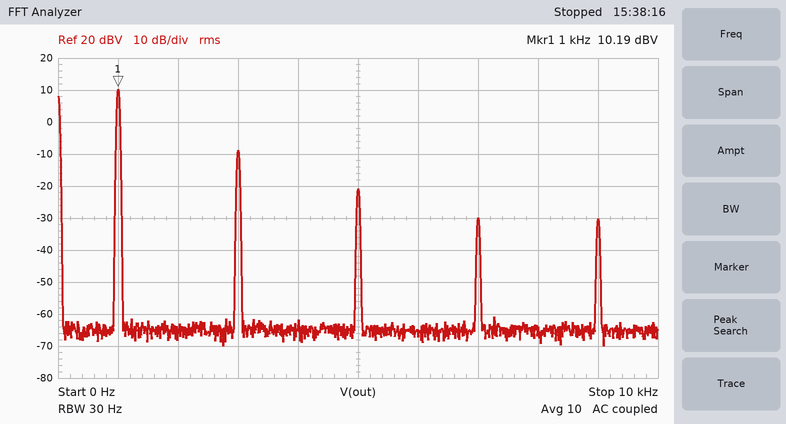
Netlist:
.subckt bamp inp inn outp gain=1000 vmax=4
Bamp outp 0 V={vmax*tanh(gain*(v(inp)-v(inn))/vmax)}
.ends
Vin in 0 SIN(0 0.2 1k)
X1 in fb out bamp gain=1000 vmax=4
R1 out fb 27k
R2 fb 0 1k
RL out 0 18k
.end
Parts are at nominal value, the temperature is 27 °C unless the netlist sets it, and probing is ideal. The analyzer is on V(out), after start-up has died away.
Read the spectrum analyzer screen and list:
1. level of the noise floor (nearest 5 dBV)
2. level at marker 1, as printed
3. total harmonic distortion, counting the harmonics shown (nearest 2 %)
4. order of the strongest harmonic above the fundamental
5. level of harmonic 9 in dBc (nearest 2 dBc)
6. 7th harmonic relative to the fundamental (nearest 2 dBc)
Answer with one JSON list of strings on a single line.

["-65 dBV", "10.19 dBV", "12 %", "3", "-40 dBc", "-40 dBc"]
